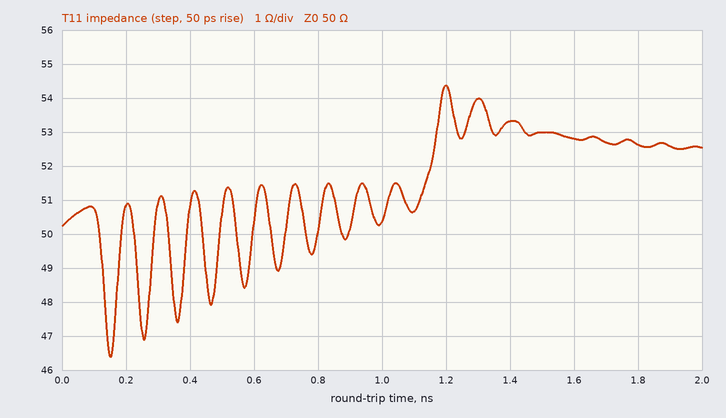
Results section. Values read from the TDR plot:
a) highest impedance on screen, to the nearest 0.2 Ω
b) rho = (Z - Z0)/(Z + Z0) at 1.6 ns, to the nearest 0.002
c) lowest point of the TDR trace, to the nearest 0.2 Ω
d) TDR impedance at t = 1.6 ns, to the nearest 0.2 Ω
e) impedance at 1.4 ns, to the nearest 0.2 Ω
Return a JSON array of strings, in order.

["54.4 Ω", "+0.028", "46.4 Ω", "52.8 Ω", "53.4 Ω"]
